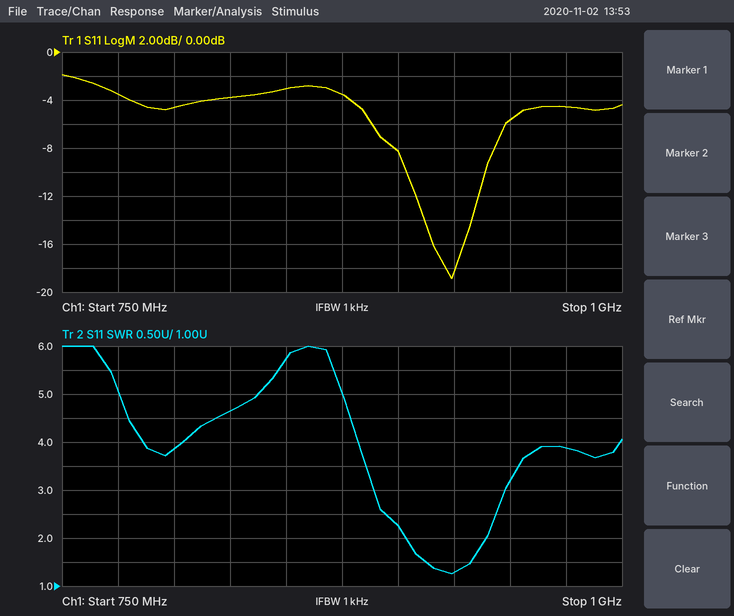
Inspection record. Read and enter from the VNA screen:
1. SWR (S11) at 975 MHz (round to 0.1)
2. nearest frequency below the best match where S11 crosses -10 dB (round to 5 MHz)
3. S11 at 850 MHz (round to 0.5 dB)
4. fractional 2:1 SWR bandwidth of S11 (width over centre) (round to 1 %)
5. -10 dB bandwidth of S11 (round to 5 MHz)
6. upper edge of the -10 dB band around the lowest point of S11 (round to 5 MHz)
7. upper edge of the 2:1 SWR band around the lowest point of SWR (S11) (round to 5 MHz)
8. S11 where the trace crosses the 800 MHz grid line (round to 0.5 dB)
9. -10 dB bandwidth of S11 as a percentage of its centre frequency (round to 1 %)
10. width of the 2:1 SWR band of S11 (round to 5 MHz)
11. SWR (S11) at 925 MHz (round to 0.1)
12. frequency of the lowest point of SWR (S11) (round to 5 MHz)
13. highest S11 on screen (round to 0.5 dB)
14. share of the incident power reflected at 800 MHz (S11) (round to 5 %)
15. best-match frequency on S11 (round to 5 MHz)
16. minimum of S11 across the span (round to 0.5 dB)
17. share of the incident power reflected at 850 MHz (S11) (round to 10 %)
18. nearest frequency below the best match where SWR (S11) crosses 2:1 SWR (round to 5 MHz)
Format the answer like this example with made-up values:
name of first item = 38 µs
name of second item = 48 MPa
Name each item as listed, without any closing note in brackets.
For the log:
SWR (S11) at 975 MHz = 3.9
nearest frequency below the best match where S11 crosses -10 dB = 905 MHz
S11 at 850 MHz = -3.0 dB
fractional 2:1 SWR bandwidth of S11 (width over centre) = 4 %
-10 dB bandwidth of S11 = 35 MHz
upper edge of the -10 dB band around the lowest point of S11 = 940 MHz
upper edge of the 2:1 SWR band around the lowest point of SWR (S11) = 940 MHz
S11 where the trace crosses the 800 MHz grid line = -4.5 dB
-10 dB bandwidth of S11 as a percentage of its centre frequency = 4 %
width of the 2:1 SWR band of S11 = 35 MHz
SWR (S11) at 925 MHz = 1.3
frequency of the lowest point of SWR (S11) = 925 MHz
highest S11 on screen = -2.0 dB
share of the incident power reflected at 800 MHz (S11) = 35 %
best-match frequency on S11 = 925 MHz
minimum of S11 across the span = -19.0 dB
share of the incident power reflected at 850 MHz (S11) = 50 %
nearest frequency below the best match where SWR (S11) crosses 2:1 SWR = 905 MHz
